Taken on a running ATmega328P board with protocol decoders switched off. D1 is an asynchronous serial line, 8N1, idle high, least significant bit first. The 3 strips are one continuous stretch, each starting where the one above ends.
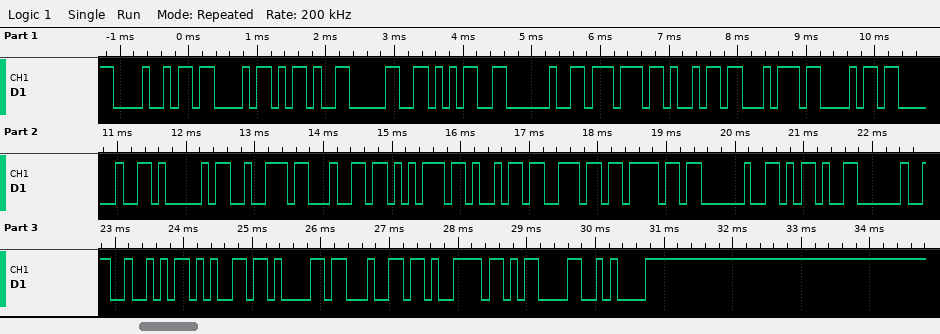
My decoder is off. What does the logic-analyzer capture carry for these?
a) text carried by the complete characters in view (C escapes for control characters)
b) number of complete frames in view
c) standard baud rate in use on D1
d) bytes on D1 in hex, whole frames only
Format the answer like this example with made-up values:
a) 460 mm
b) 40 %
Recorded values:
a) "HC-05 with Arduino - Ready\r\n"
b) 28
c) 9600 baud
d) 48 43 2D 30 35 20 77 69 74 68 20 41 72 64 75 69 6E 6F 20 2D 20 52 65 61 64 79 0D 0A
